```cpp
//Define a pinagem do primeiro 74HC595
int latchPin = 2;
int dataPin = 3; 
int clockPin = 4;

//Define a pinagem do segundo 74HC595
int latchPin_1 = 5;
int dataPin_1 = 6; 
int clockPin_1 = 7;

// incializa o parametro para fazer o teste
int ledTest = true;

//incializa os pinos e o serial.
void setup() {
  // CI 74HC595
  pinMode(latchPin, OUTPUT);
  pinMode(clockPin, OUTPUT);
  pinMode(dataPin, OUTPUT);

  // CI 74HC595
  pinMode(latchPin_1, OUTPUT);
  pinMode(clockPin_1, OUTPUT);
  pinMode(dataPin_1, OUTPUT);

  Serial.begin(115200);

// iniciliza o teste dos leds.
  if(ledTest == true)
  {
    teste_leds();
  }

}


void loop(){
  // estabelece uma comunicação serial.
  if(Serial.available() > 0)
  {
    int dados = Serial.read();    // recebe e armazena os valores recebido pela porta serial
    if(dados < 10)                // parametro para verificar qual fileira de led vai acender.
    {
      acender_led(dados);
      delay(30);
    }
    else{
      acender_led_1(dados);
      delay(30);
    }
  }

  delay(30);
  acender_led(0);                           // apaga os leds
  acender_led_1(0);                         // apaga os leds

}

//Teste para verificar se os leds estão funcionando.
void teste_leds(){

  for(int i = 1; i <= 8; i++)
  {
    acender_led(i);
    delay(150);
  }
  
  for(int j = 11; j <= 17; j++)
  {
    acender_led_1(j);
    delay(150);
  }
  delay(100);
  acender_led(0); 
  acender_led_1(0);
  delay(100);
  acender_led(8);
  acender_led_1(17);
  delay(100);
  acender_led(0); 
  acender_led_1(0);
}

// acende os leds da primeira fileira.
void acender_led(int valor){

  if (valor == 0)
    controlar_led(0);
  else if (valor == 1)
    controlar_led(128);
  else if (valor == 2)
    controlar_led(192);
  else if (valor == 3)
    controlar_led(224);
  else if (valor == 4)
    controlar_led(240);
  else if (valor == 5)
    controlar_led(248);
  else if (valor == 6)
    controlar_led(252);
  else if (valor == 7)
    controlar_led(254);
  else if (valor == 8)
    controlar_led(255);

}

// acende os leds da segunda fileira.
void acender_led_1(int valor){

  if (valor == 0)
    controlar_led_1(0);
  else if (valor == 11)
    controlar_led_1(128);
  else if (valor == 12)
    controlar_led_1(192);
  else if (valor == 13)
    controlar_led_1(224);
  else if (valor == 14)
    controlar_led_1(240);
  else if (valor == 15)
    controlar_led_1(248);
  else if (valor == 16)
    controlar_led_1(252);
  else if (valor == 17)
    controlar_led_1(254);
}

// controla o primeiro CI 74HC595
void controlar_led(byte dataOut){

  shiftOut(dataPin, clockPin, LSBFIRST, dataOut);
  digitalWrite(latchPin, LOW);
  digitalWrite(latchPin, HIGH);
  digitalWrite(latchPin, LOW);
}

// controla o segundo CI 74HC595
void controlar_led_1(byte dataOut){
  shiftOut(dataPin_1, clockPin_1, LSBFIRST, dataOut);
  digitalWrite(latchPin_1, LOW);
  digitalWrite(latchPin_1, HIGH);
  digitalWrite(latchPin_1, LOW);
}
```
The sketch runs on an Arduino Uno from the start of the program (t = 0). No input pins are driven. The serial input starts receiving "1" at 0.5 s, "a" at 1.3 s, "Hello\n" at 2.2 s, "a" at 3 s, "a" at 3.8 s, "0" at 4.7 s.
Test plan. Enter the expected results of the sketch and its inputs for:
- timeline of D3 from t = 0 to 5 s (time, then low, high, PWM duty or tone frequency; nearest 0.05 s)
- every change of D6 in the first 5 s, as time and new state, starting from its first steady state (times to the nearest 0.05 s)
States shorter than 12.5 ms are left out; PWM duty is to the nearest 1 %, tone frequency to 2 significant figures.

0 s high; 2.35 s low; 2.45 s high; 2.55 s low
0 s low; 1.2 s high; 2.35 s low; 2.45 s high; 2.55 s low
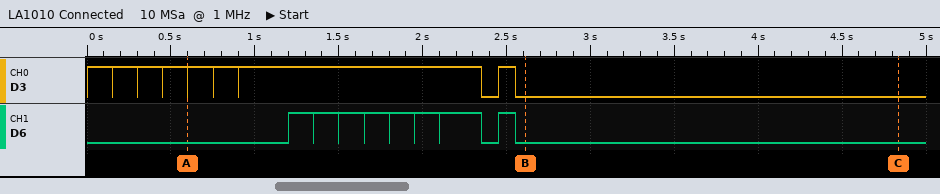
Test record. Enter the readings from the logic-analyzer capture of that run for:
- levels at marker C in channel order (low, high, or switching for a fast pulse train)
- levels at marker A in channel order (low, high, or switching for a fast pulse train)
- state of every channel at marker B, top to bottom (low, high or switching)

D3 low, D6 low
D3 high, D6 low
D3 low, D6 low
